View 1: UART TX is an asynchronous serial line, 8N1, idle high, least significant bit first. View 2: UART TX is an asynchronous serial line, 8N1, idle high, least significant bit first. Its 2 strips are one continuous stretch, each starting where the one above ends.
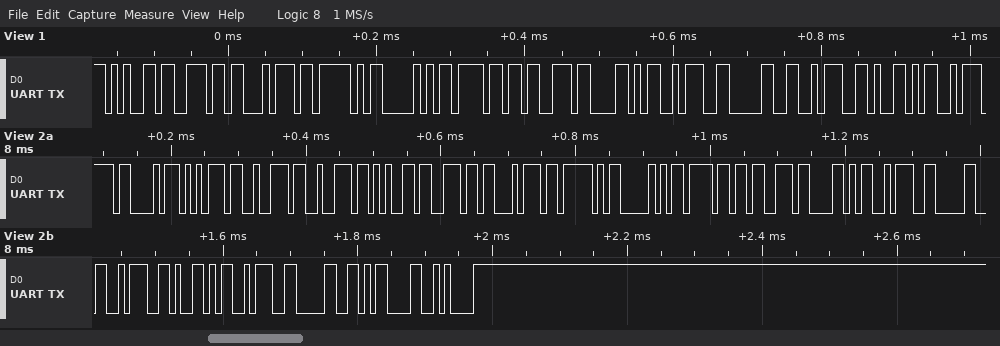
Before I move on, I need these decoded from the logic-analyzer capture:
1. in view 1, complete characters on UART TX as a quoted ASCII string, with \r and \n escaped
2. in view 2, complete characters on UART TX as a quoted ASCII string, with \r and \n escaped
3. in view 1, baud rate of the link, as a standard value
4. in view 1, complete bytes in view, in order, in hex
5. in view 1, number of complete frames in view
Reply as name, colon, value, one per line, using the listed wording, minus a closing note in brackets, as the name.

in view 1, complete characters on UART TX as a quoted ASCII string, with \r and \n escaped: "ent_PosX:0:Y"
in view 2, complete characters on UART TX as a quoted ASCII string, with \r and \n escaped: "Current_PosX:0:Y:0\r\n"
in view 1, baud rate of the link, as a standard value: 115200 baud
in view 1, complete bytes in view, in order, in hex: 65 6E 74 5F 50 6F 73 58 3A 30 3A 59
in view 1, number of complete frames in view: 12
